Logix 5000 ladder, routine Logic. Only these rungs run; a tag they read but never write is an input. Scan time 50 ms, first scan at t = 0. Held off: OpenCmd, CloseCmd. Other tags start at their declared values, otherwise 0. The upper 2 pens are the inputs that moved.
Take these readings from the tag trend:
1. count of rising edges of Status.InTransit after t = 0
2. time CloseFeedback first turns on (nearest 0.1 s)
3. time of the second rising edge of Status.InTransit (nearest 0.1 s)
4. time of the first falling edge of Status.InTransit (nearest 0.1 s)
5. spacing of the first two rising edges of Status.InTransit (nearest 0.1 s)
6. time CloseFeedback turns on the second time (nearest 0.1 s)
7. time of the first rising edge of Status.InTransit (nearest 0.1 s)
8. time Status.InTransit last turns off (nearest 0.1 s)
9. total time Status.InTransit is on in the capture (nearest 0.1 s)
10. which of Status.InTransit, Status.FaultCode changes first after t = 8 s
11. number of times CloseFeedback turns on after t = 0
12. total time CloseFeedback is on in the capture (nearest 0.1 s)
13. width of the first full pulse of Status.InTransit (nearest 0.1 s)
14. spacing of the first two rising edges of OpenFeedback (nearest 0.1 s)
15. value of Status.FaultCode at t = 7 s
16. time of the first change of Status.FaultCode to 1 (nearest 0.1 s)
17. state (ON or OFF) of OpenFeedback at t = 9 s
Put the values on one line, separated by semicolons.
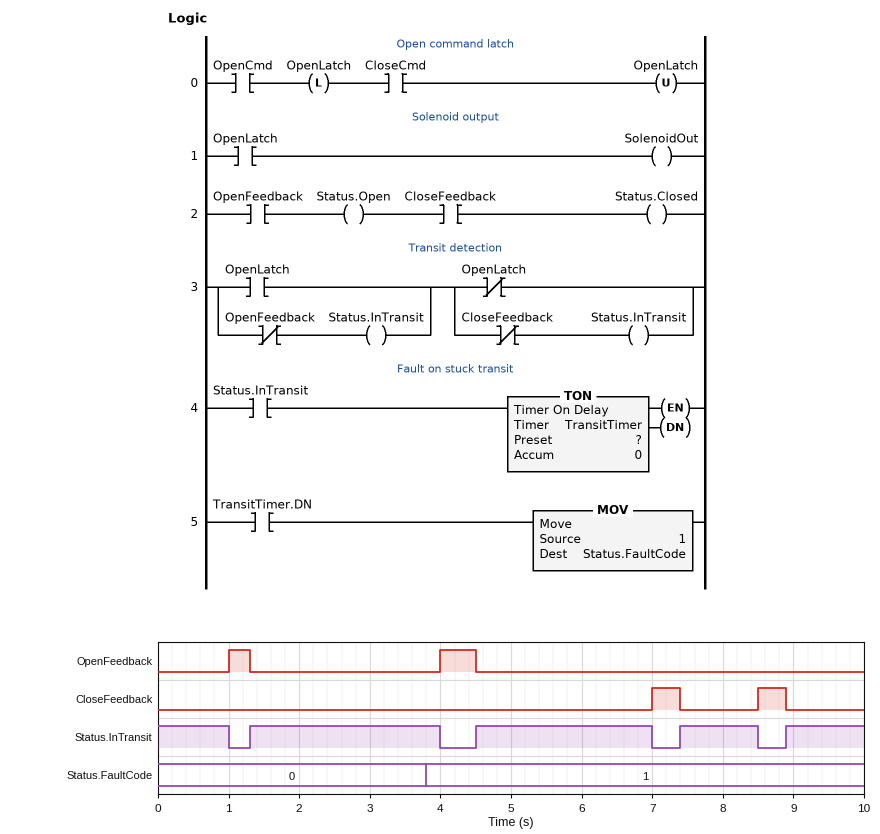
4; 7.0 s; 4.5 s; 1.0 s; 3.2 s; 8.5 s; 1.3 s; 8.5 s; 8.4 s; Status.InTransit; 2; 0.8 s; 2.7 s; 3.0 s; 1; 3.8 s; OFF
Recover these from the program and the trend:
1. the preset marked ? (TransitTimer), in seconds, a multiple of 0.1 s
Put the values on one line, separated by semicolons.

2.5 s
